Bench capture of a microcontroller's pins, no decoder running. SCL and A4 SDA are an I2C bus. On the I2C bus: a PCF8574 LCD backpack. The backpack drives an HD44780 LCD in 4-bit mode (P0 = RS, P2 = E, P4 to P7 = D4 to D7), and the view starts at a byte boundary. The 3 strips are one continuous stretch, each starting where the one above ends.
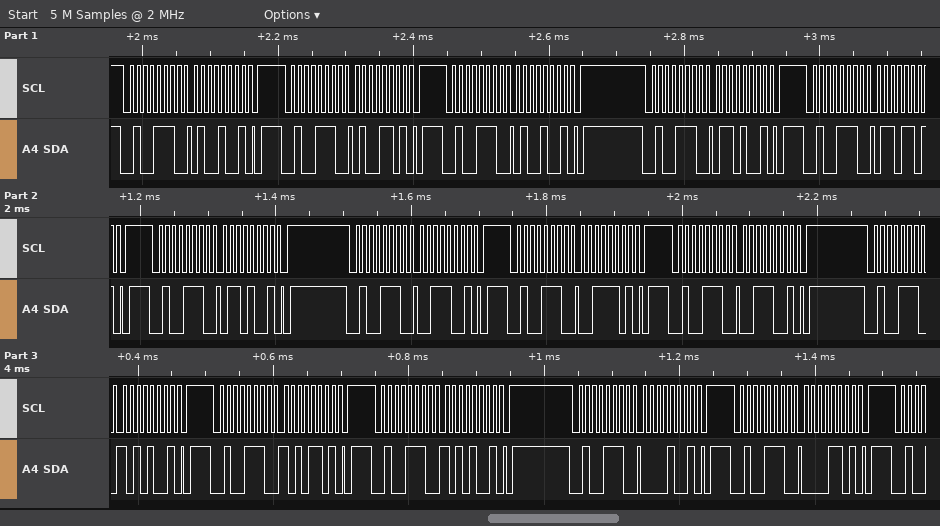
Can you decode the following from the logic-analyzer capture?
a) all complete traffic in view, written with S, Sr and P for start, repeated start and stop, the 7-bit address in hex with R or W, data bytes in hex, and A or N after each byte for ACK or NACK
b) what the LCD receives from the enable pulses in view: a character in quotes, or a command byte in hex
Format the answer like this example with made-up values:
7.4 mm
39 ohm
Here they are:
S 27W A 49 A P S 27W A 4D A P S 27W A 49 A P S 27W A 69 A P S 27W A 6D A P S 27W A 69 A P S 27W A 39 A P S 27W A 3D A P S 27W A 39 A P S 27W A A9 A P S 27W A AD A P S 27W A A9 A P S 27W A 09 A P S 27W A 0D A P
'F' ':'
